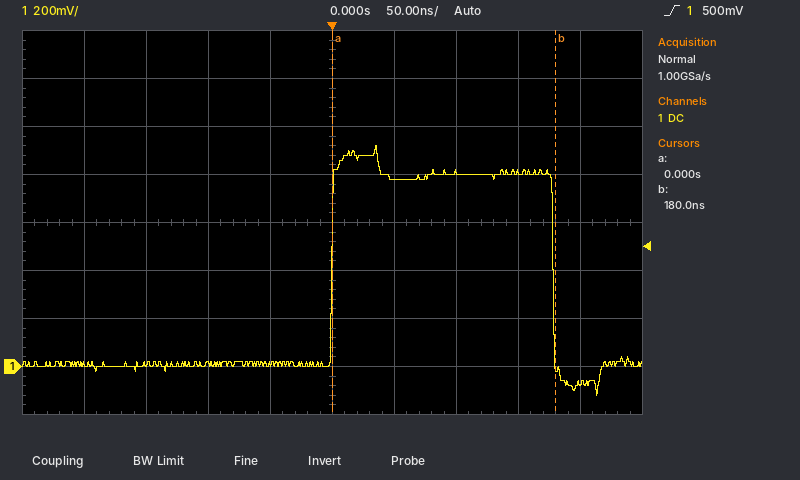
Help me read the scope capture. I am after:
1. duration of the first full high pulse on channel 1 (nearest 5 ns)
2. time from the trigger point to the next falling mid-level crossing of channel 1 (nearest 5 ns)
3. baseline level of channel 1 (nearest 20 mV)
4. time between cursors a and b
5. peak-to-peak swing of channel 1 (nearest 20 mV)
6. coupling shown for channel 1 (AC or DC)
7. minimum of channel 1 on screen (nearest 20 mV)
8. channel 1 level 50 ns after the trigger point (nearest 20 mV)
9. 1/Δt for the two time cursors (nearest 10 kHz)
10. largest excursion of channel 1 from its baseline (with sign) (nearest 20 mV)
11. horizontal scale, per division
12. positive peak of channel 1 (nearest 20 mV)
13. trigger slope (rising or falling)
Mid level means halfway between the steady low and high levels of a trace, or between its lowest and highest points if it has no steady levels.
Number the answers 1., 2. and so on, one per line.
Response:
1. 180 ns
2. 180 ns
3. 0 mV
4. 180 ns
5. 1.04 V
6. DC
7. -120 mV
8. 780 mV
9. 5.56 MHz
10. +920 mV
11. 50 ns
12. 920 mV
13. rising
